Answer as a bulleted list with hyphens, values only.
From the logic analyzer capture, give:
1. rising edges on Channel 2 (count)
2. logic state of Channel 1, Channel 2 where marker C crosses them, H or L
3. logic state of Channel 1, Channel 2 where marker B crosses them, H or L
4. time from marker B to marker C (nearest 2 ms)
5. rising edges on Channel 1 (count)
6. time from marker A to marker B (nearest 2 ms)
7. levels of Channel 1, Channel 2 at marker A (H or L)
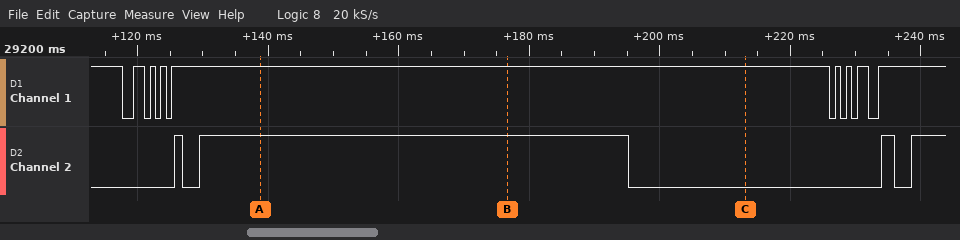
- 4
- Channel 1=H, Channel 2=L
- Channel 1=H, Channel 2=H
- 36 ms
- 8
- 38 ms
- Channel 1=H, Channel 2=H
